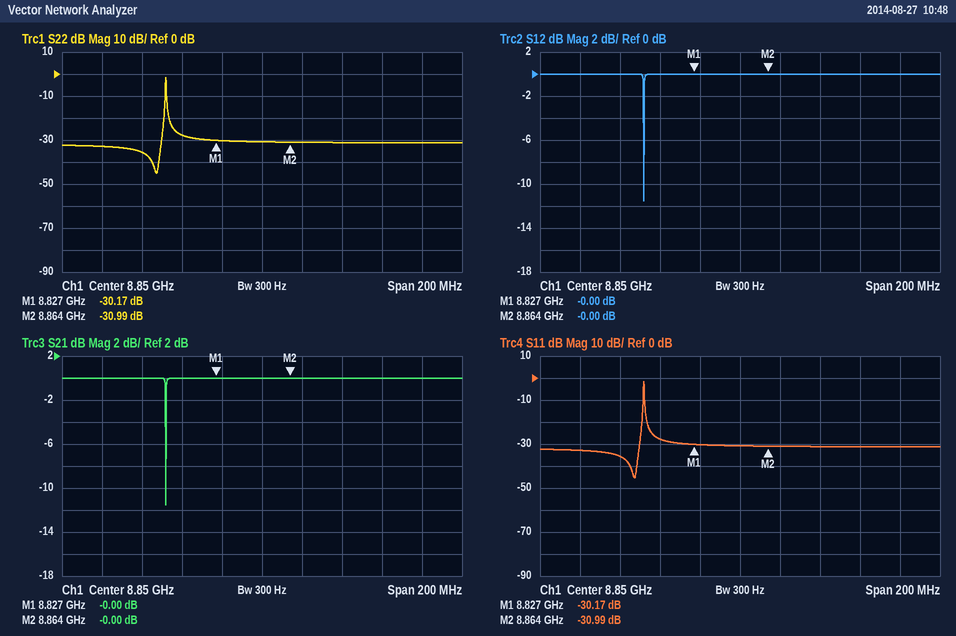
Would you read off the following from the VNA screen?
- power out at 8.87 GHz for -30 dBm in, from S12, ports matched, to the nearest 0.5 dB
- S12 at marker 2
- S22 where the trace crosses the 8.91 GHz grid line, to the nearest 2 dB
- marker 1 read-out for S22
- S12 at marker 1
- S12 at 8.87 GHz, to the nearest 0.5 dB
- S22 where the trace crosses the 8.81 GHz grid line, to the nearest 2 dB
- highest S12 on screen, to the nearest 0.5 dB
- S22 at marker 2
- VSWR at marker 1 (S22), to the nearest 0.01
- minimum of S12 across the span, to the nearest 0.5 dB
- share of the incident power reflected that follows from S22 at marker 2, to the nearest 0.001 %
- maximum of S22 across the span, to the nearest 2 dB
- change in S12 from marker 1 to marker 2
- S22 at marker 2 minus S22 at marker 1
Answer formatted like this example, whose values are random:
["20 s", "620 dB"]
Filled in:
["-30.0 dBm", "-0.00 dB", "-32 dB", "-30.17 dB", "-0.00 dB", "0.0 dB", "-28 dB", "0.0 dB", "-30.99 dB", "1.06", "-11.5 dB", "0.080 %", "-2 dB", "0.00 dB", "-0.82 dB"]
